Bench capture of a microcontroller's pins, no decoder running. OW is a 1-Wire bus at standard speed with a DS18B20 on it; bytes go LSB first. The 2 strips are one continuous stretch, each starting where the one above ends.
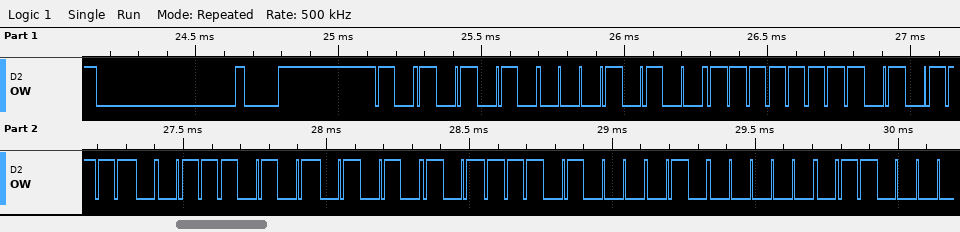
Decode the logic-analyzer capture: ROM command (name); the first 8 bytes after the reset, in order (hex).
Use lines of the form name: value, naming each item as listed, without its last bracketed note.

ROM command: Match ROM
the first 8 bytes after the reset, in order: 55 28 FF 7A AE AA 17 02
